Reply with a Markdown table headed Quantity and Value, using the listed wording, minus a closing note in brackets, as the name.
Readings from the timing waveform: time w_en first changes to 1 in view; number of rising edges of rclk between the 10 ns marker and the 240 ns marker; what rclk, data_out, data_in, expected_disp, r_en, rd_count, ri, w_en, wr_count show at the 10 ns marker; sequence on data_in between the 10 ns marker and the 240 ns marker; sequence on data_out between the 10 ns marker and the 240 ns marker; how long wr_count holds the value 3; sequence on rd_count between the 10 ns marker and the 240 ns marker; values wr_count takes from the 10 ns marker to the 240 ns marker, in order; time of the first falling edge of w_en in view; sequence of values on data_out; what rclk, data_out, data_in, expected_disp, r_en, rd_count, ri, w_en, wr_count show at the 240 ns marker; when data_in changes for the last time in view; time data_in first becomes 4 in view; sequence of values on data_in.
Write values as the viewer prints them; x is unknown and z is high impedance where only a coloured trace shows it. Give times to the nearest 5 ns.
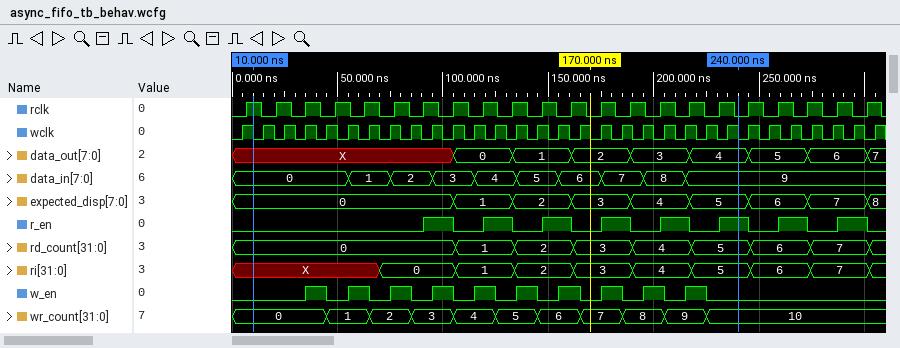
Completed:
| Quantity | Value |
|---|---|
| time w_en first changes to 1 in view | 35 ns |
| number of rising edges of rclk between the 10 ns marker and the 240 ns marker | 16 |
| what rclk, data_out, data_in, expected_disp, r_en, rd_count, ri, w_en, wr_count show at the 10 ns marker | rclk=1, data_out=X, data_in=0, expected_disp=0, r_en=0, rd_count=0, ri=X, w_en=0, wr_count=0 |
| sequence on data_in between the 10 ns marker and the 240 ns marker | 0, 1, 2, 3, 4, 5, 6, 7, 8, 9 |
| sequence on data_out between the 10 ns marker and the 240 ns marker | X, 0, 1, 2, 3, 4 |
| how long wr_count holds the value 3 | 20 ns |
| sequence on rd_count between the 10 ns marker and the 240 ns marker | 0, 1, 2, 3, 4, 5 |
| values wr_count takes from the 10 ns marker to the 240 ns marker, in order | 0, 1, 2, 3, 4, 5, 6, 7, 8, 9, 10 |
| time of the first falling edge of w_en in view | 45 ns |
| sequence of values on data_out | X, 0, 1, 2, 3, 4, 5, 6, 7 |
| what rclk, data_out, data_in, expected_disp, r_en, rd_count, ri, w_en, wr_count show at the 240 ns marker | rclk=0, data_out=4, data_in=9, expected_disp=5, r_en=1, rd_count=5, ri=5, w_en=0, wr_count=10 |
| when data_in changes for the last time in view | 215 ns |
| time data_in first becomes 4 in view | 115 ns |
| sequence of values on data_in | 0, 1, 2, 3, 4, 5, 6, 7, 8, 9 |
